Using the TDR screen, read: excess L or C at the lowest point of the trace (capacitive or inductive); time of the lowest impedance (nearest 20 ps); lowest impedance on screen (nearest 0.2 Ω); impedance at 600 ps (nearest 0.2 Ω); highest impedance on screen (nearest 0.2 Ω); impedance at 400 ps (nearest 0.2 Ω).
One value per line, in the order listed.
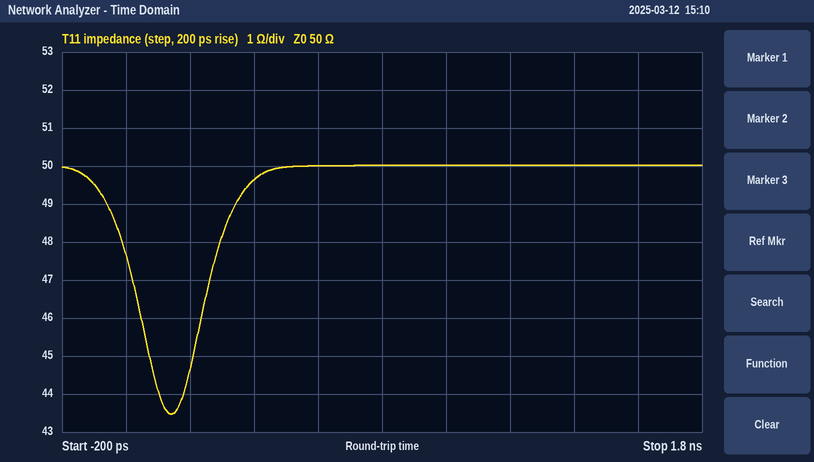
capacitive
140 ps
43.4 Ω
50.0 Ω
50.0 Ω
49.6 Ω
